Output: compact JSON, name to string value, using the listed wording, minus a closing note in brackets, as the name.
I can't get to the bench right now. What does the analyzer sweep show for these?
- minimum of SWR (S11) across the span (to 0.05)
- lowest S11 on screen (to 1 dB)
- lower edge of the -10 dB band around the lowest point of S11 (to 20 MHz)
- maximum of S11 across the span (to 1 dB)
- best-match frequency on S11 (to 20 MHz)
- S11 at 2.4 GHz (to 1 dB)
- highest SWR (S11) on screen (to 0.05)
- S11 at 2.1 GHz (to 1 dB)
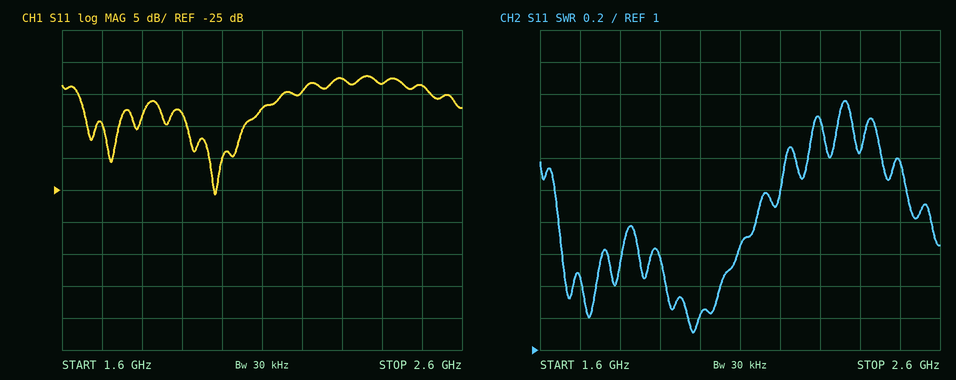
{"minimum of SWR (S11) across the span": "1.10", "lowest S11 on screen": "-26 dB", "lower edge of the -10 dB band around the lowest point of S11": "1.64 GHz", "maximum of S11 across the span": "-7 dB", "best-match frequency on S11": "1.98 GHz", "S11 at 2.4 GHz": "-8 dB", "highest SWR (S11) on screen": "2.55", "S11 at 2.1 GHz": "-12 dB"}
